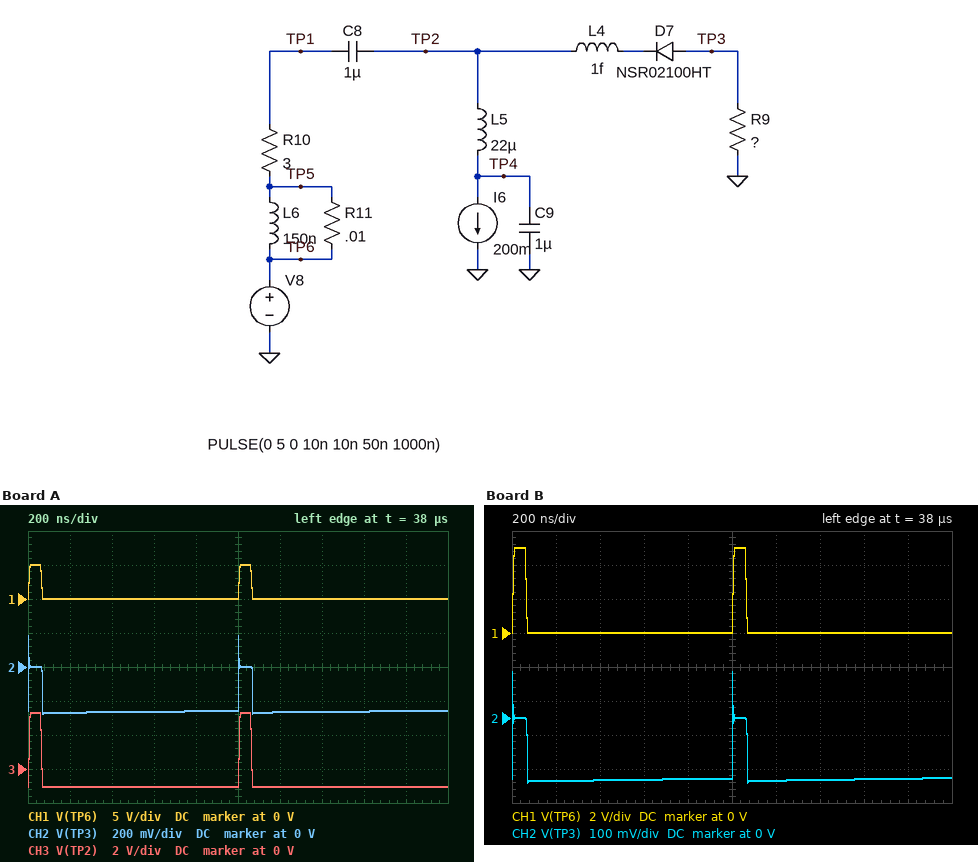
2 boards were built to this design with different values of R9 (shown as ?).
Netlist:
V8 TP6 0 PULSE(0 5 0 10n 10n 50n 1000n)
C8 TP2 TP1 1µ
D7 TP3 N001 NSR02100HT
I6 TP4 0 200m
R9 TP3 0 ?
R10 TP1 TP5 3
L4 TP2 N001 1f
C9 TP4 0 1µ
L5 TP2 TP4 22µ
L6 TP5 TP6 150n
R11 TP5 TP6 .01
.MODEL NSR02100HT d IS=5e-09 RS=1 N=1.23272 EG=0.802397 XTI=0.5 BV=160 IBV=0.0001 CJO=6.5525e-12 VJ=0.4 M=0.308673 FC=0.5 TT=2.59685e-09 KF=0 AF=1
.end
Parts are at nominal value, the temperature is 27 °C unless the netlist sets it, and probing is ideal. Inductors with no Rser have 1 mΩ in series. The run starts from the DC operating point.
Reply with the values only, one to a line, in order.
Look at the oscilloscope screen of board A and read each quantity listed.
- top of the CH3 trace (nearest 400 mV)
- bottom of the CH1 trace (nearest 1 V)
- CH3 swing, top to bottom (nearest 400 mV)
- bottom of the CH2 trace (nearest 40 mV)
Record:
3.2 V
0 V
4.4 V
-280 mV
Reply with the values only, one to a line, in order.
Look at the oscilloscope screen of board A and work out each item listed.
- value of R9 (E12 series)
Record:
1.2 Ω
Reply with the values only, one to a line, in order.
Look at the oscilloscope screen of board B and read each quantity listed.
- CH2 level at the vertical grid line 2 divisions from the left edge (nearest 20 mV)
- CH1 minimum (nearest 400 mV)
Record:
-180 mV
0 V
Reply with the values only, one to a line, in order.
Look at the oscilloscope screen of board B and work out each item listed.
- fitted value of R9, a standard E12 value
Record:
0.82 Ω
